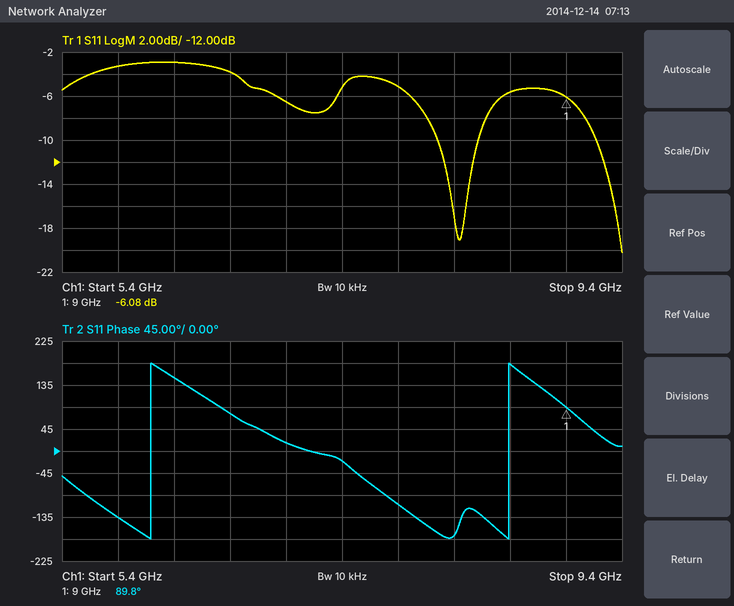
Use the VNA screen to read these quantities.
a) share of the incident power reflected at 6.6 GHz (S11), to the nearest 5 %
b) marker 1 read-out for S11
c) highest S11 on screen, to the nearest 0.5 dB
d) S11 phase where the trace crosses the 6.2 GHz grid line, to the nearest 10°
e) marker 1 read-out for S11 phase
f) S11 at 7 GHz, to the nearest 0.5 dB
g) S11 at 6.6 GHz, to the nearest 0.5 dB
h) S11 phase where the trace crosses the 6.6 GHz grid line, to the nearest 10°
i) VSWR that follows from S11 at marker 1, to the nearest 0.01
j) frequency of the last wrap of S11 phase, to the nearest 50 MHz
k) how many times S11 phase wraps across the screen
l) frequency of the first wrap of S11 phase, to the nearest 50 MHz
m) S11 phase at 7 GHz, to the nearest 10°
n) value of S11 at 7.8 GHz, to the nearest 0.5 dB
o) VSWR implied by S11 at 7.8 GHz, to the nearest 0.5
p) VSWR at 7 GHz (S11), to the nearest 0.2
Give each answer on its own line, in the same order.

40 %
-6.08 dB
-3.0 dB
150°
89.8°
-6.5 dB
-4.0 dB
80°
2.97
8.60 GHz
2
6.05 GHz
20°
-5.0 dB
3.5
2.8
